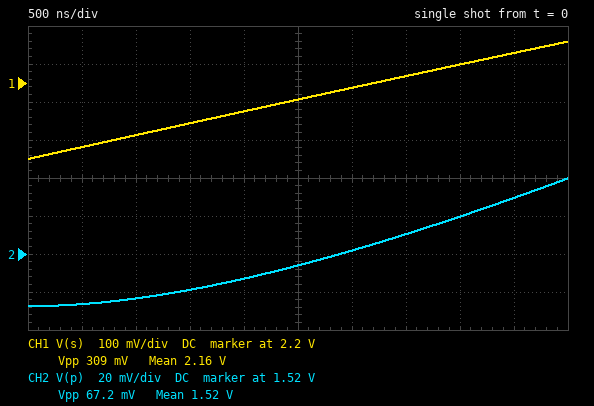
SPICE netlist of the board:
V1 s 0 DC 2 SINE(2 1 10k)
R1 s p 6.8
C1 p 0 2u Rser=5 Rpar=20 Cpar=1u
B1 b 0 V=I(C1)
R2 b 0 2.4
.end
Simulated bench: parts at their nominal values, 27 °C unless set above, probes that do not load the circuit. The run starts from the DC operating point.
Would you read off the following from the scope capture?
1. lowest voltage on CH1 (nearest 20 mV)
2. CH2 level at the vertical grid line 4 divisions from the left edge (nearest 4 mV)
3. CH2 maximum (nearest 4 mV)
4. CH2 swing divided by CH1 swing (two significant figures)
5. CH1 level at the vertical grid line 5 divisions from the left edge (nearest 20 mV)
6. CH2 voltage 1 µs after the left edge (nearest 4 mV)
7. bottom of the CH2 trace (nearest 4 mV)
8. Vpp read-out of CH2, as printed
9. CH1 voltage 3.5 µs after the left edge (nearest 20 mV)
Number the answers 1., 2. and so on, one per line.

1. 2.00 V
2. 1.508 V
3. 1.560 V
4. 0.22
5. 2.16 V
6. 1.496 V
7. 1.492 V
8. 67.2 mV
9. 2.22 V
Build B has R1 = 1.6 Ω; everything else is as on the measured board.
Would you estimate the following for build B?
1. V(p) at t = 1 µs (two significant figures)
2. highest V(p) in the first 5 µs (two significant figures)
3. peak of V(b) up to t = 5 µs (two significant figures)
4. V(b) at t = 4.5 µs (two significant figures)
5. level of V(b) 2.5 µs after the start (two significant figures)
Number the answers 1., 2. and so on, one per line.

1. 1.9 V
2. 2.0 V
3. 29 mV
4. 26 mV
5. 12 mV
